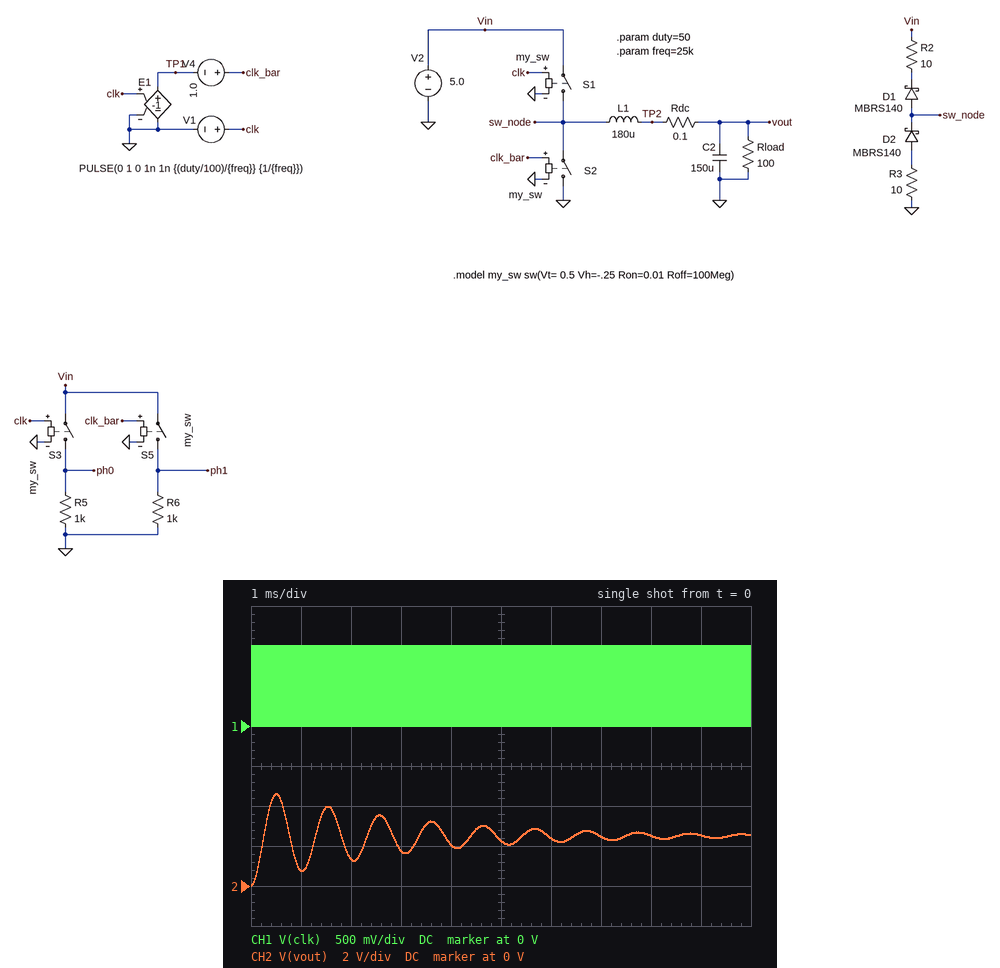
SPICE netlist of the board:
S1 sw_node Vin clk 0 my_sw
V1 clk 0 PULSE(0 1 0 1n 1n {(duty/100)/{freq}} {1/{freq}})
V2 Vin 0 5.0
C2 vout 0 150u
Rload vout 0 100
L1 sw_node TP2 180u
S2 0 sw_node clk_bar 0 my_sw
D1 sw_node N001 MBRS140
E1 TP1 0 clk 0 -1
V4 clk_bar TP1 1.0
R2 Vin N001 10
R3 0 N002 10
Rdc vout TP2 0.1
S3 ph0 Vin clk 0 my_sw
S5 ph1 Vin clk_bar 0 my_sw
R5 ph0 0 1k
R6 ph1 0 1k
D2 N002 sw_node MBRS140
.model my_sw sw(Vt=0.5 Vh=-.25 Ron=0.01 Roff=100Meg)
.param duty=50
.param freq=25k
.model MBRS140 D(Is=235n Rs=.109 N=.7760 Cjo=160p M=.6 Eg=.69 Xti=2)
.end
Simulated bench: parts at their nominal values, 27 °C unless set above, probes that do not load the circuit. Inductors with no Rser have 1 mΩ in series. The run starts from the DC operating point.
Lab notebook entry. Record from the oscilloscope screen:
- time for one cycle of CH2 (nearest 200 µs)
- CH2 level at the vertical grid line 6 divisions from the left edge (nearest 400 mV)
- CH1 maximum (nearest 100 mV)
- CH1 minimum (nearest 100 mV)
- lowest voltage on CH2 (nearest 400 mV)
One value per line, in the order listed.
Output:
1.0 ms
2.4 V
1.0 V
0 V
0 V
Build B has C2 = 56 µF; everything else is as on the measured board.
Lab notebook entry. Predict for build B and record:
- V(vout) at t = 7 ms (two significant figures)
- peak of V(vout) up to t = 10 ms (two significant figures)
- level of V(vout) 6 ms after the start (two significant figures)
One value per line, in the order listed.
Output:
2.4 V
4.7 V
2.7 V
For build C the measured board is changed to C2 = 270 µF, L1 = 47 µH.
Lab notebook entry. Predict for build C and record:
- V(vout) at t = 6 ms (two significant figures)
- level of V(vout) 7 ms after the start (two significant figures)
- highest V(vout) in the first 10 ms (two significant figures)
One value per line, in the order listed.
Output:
2.5 V
2.5 V
4.1 V
